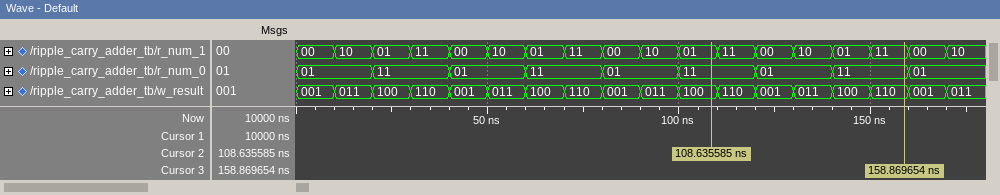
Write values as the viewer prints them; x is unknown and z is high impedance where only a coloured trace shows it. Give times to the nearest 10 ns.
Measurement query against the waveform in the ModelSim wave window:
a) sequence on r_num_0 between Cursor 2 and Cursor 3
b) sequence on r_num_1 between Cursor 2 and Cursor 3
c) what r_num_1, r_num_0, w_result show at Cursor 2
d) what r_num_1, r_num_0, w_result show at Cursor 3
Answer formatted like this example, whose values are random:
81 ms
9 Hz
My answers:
11, 01, 11
01, 11, 00, 10, 01, 11
r_num_1=01, r_num_0=11, w_result=100
r_num_1=11, r_num_0=11, w_result=110
